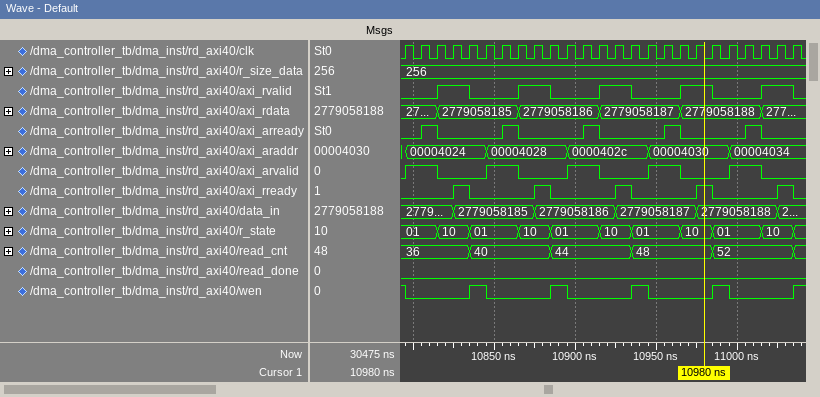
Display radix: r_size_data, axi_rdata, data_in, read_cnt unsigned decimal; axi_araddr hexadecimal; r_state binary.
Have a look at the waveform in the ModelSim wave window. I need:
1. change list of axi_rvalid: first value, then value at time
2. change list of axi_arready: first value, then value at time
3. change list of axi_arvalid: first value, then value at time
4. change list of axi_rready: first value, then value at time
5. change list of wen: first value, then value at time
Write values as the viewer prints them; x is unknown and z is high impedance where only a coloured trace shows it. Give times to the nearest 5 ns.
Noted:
0, 1 at 10815 ns, 0 at 10835 ns, 1 at 10865 ns, 0 at 10885 ns, 1 at 10915 ns, 0 at 10935 ns, 1 at 10965 ns, 0 at 10985 ns, 1 at 11015 ns, 0 at 11035 ns
0, 1 at 10805 ns, 0 at 10815 ns, 1 at 10855 ns, 0 at 10865 ns, 1 at 10905 ns, 0 at 10915 ns, 1 at 10955 ns, 0 at 10965 ns, 1 at 11005 ns, 0 at 11015 ns
0, 1 at 10795 ns, 0 at 10815 ns, 1 at 10845 ns, 0 at 10865 ns, 1 at 10895 ns, 0 at 10915 ns, 1 at 10945 ns, 0 at 10965 ns, 1 at 10995 ns, 0 at 11015 ns
0, 1 at 10825 ns, 0 at 10835 ns, 1 at 10875 ns, 0 at 10885 ns, 1 at 10925 ns, 0 at 10935 ns, 1 at 10975 ns, 0 at 10985 ns, 1 at 11025 ns, 0 at 11035 ns
1, 0 at 10795 ns, 1 at 10835 ns, 0 at 10845 ns, 1 at 10885 ns, 0 at 10895 ns, 1 at 10935 ns, 0 at 10945 ns, 1 at 10985 ns, 0 at 10995 ns, 1 at 11035 ns
